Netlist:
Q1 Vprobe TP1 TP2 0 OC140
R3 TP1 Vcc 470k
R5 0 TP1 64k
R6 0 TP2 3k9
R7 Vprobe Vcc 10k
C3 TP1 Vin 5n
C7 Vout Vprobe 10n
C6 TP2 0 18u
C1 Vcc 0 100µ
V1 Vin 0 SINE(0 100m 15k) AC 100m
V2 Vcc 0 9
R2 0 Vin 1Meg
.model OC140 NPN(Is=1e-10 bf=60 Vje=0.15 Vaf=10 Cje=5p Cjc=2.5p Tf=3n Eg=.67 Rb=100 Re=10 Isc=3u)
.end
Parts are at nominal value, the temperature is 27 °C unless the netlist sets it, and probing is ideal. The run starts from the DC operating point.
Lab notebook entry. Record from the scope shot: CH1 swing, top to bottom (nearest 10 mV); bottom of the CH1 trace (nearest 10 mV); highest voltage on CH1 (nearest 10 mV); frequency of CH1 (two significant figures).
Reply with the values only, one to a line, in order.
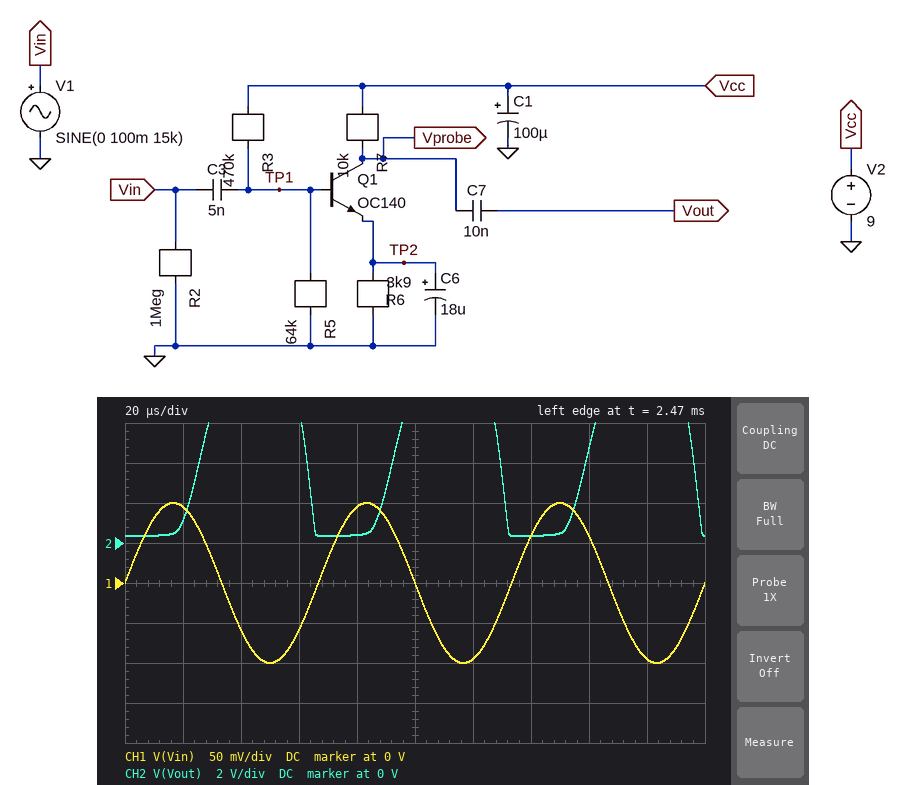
200 mV
-100 mV
100 mV
15 kHz
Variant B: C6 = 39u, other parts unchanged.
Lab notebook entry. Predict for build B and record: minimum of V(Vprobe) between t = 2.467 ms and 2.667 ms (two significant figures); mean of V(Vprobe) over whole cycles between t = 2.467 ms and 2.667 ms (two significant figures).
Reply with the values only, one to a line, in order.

310 mV
4.7 V
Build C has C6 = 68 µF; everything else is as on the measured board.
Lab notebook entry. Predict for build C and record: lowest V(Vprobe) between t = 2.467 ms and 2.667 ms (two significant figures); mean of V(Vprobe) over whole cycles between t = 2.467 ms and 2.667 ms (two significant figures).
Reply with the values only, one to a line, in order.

300 mV
4.6 V
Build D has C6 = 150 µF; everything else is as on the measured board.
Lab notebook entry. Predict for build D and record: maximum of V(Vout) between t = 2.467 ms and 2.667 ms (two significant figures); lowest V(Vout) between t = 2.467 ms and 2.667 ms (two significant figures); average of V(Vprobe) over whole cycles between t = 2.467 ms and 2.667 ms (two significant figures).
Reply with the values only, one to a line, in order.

8.8 V
290 mV
4.6 V
